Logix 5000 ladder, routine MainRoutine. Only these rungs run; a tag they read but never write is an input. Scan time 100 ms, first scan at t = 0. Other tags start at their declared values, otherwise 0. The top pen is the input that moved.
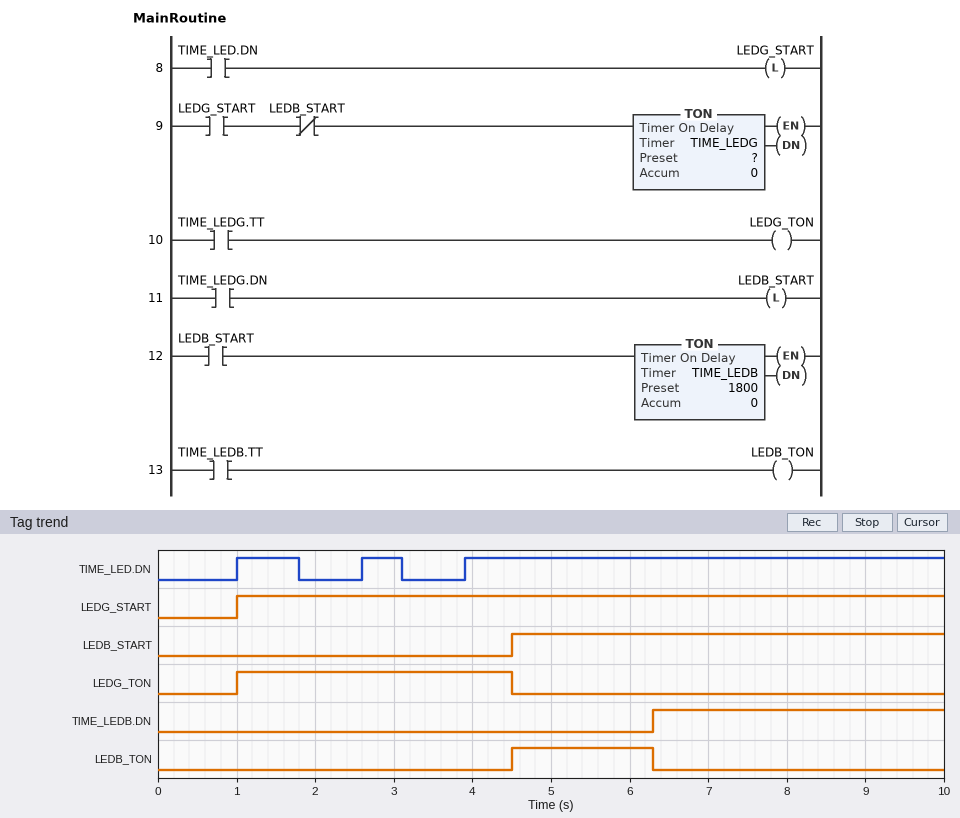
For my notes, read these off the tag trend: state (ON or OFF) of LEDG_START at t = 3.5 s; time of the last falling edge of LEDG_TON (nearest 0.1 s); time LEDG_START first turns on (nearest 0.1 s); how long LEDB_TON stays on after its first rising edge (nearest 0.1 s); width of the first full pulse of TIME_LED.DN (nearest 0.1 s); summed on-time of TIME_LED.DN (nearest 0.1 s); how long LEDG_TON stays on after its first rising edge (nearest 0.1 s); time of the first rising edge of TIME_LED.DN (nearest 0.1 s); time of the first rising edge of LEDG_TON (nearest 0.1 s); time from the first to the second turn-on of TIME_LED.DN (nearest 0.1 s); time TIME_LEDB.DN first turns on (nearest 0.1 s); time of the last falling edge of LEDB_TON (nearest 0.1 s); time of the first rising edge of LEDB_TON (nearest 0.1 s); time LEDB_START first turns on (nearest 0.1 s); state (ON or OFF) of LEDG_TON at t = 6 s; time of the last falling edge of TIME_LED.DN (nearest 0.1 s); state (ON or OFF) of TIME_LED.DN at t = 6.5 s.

ON
4.5 s
1.0 s
1.8 s
0.8 s
7.4 s
3.5 s
1.0 s
1.0 s
1.6 s
6.3 s
6.3 s
4.5 s
4.5 s
OFF
3.1 s
ON
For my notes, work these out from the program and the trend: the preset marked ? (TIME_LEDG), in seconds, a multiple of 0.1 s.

3.5 s
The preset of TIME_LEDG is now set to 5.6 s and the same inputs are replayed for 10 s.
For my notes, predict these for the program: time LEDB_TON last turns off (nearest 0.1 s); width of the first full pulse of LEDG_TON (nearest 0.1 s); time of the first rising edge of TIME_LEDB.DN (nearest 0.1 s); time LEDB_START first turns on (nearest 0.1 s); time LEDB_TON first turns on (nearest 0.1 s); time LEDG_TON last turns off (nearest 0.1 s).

8.4 s
5.6 s
8.4 s
6.6 s
6.6 s
6.6 s
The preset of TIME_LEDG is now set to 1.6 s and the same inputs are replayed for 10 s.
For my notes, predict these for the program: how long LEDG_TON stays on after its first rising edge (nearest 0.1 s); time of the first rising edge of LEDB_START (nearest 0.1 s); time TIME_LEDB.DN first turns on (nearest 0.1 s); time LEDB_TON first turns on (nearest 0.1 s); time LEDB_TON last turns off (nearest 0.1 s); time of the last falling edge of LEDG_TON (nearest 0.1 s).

1.6 s
2.6 s
4.4 s
2.6 s
4.4 s
2.6 s
